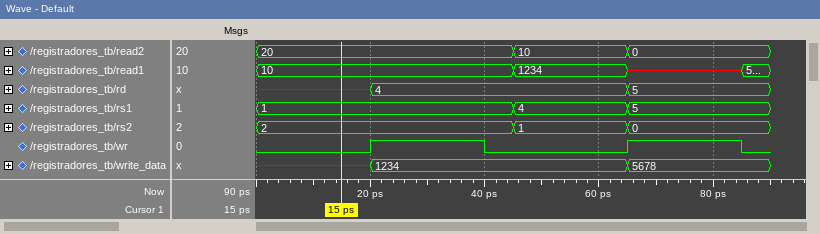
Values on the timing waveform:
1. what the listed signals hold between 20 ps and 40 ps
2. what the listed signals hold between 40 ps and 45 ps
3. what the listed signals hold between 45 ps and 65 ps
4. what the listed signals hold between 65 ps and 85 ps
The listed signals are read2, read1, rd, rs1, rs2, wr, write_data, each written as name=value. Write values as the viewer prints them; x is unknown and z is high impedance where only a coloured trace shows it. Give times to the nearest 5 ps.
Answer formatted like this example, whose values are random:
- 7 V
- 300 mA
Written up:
- read2=20, read1=10, rd=4, rs1=1, rs2=2, wr=1, write_data=1234
- read2=20, read1=10, rd=4, rs1=1, rs2=2, wr=0, write_data=1234
- read2=10, read1=1234, rd=4, rs1=4, rs2=1, wr=0, write_data=1234
- read2=0, read1=x, rd=5, rs1=5, rs2=0, wr=1, write_data=5678
